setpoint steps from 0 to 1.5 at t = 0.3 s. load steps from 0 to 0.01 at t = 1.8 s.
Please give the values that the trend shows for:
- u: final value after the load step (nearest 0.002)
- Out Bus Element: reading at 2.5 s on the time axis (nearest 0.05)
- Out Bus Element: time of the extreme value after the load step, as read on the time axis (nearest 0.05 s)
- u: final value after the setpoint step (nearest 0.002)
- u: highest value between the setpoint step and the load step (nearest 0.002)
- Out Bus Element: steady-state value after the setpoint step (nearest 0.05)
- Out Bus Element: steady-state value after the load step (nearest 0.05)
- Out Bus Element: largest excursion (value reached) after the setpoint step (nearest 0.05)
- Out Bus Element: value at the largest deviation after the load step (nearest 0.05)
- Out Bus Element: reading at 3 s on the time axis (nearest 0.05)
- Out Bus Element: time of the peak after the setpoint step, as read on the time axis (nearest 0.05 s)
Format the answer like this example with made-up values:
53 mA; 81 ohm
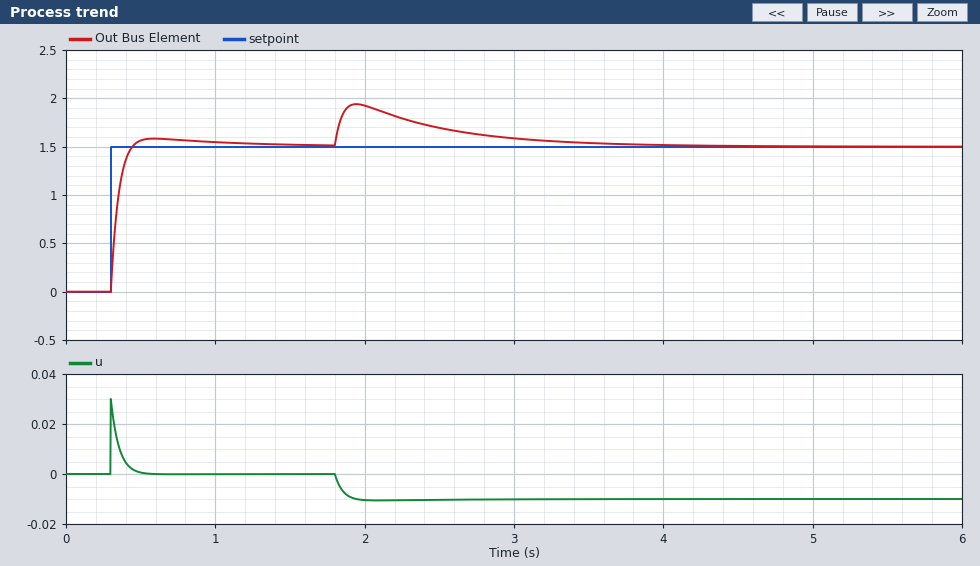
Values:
-0.010; 1.70; 1.95 s; 0.000; 0.030; 1.50; 1.50; 1.60; 1.95; 1.60; 0.60 s
